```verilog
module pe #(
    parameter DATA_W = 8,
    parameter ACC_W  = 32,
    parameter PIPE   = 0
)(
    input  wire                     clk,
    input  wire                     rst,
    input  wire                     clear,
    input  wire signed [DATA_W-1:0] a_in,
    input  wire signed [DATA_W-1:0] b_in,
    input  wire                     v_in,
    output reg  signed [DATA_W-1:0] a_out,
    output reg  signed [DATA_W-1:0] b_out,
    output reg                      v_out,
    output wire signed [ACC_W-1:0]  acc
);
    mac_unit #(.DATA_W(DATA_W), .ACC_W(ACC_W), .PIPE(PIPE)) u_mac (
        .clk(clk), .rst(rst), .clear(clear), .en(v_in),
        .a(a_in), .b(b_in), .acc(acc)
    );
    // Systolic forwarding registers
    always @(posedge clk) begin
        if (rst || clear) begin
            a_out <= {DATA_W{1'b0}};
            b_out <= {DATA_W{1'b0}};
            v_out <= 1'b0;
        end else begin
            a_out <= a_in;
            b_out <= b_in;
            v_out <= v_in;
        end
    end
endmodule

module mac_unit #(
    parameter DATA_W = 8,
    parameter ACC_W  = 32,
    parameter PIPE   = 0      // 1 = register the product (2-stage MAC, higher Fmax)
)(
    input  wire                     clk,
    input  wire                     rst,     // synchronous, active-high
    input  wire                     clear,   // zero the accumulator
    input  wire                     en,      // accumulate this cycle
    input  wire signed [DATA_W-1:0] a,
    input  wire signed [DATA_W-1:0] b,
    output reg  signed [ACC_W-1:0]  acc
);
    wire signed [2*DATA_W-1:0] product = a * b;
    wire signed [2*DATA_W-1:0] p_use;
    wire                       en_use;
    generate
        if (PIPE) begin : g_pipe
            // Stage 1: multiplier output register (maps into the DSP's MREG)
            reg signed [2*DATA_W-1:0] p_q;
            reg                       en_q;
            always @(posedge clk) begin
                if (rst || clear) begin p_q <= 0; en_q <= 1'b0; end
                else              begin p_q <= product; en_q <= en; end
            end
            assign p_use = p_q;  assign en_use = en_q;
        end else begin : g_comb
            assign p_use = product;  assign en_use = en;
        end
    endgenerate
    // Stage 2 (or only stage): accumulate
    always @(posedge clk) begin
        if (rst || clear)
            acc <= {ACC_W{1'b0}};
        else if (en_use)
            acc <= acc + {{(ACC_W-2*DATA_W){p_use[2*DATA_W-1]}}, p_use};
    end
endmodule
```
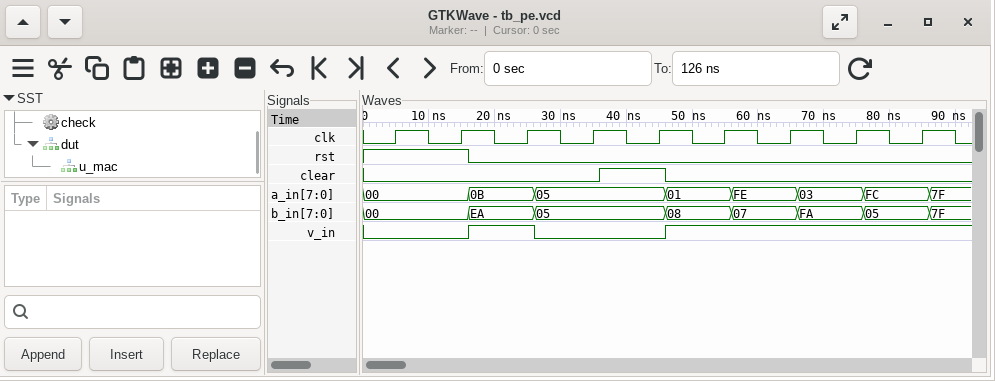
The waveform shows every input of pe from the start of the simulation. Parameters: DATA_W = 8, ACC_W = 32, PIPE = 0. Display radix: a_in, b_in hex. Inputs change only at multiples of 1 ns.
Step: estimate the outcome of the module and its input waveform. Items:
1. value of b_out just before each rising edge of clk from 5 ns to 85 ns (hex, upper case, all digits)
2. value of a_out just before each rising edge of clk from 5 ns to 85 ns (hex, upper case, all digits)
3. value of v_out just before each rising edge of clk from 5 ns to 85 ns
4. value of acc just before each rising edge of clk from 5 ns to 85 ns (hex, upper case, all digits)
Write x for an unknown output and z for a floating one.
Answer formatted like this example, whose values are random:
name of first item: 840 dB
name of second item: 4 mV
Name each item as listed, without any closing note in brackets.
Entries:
value of b_out just before each rising edge of clk from 5 ns to 85 ns: x, 00, 00, EA, 05, 00, 08, 07, FA
value of a_out just before each rising edge of clk from 5 ns to 85 ns: x, 00, 00, 0B, 05, 00, 01, FE, 03
value of v_out just before each rising edge of clk from 5 ns to 85 ns: x 0 0 1 0 0 1 1 1
value of acc just before each rising edge of clk from 5 ns to 85 ns: x, 00000000, 00000000, FFFFFF0E, FFFFFF0E, 00000000, 00000008, FFFFFFFA, FFFFFFE8
